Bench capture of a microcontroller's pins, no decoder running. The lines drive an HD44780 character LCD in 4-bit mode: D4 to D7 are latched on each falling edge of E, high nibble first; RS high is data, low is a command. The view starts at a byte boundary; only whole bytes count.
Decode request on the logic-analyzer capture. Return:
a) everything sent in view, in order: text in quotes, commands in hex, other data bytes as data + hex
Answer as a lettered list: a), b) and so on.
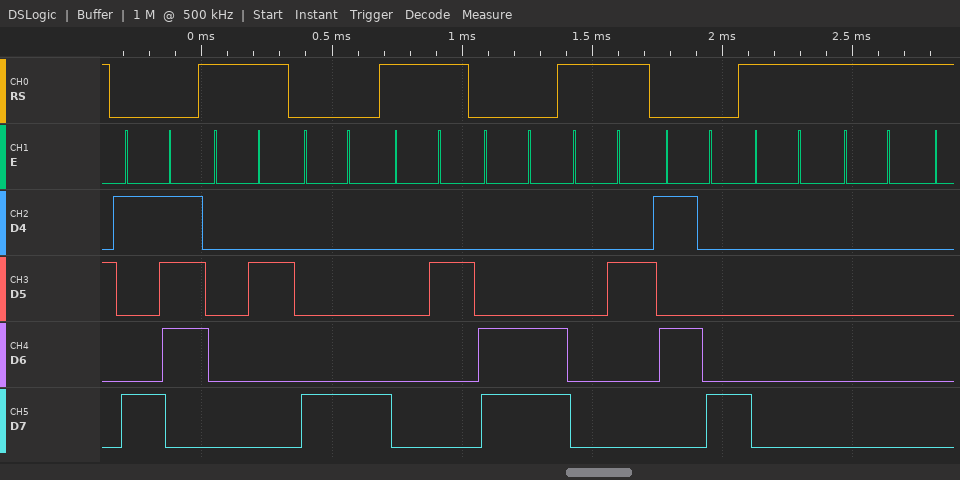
a) 0x97 data 02 0x88 data 02 0xCC data 02 0x58 data 00 00
